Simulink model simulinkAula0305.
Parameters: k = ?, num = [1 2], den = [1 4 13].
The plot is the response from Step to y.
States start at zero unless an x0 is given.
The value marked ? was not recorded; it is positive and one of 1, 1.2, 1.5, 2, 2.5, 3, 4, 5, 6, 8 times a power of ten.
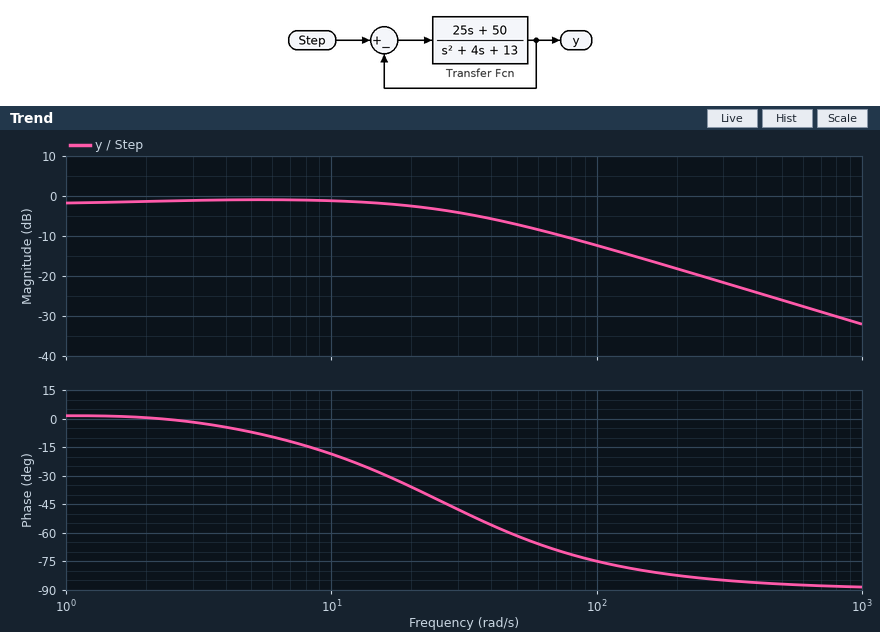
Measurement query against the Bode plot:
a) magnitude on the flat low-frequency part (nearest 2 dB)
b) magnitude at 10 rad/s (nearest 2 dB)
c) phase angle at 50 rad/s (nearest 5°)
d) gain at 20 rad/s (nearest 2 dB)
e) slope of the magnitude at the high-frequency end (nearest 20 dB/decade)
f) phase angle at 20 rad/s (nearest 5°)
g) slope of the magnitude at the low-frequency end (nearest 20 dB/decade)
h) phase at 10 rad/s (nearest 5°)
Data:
-2 dB
-2 dB
-60°
-2 dB
-20 dB/decade
-35°
0 dB/decade
-20°
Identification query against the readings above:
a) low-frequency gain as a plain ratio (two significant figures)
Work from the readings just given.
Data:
0.79
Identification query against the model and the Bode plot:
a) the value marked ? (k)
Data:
25
